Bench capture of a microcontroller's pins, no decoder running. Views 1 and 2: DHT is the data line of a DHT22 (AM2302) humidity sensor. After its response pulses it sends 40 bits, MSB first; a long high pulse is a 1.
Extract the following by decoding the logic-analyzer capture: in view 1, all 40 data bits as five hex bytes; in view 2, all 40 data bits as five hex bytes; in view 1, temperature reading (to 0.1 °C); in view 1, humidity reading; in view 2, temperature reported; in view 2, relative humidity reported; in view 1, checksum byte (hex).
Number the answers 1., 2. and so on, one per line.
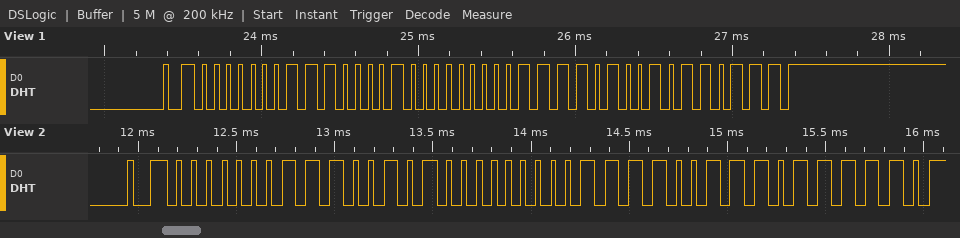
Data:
1. 01 C2 00 F4 B7
2. 01 CA 00 F3 BE
3. 24.4 °C
4. 45.0 %
5. 24.3 °C
6. 45.8 %
7. 0xB7
